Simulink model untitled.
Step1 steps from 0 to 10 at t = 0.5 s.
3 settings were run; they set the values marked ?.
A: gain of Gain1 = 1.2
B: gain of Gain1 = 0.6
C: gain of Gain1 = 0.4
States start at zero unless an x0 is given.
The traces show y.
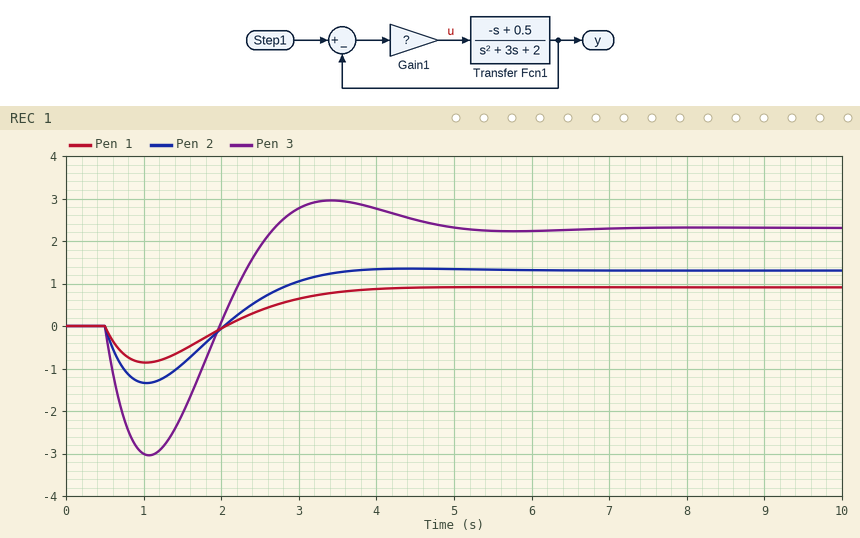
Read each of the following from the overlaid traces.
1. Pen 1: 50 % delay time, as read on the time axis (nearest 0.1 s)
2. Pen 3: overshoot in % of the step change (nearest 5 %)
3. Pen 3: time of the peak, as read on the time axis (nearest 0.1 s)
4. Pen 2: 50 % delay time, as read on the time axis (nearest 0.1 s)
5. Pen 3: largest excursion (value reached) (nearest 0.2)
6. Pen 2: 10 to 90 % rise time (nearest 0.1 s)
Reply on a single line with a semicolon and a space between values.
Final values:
2.6 s; 30 %; 3.4 s; 2.5 s; 3.0; 1.1 s
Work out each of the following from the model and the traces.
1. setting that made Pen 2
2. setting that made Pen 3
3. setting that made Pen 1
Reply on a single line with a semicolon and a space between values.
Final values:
B; A; C
